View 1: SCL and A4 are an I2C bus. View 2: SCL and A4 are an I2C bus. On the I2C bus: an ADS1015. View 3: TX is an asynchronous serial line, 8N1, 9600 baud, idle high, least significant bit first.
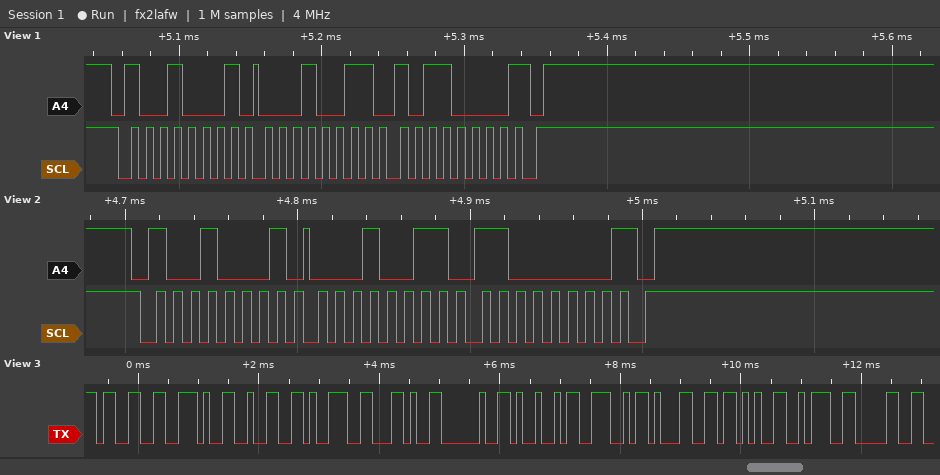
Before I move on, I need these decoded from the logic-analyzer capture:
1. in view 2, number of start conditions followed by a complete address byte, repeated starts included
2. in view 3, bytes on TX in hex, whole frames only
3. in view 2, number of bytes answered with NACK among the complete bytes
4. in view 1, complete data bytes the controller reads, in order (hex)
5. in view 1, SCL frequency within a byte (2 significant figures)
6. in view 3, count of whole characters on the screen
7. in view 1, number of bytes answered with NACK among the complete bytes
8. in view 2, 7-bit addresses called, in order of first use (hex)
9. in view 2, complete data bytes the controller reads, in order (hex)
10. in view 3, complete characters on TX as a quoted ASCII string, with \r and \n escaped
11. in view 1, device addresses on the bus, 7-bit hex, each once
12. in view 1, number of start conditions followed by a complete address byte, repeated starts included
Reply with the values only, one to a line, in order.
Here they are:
1
0x33 0x2E 0x32 0x39 0x2C 0x20 0x49 0x4E 0x31 0x2B 0x3A 0x30
1
13 B0
100 kHz
12
1
0x48
13 C0
"3.29, IN1+:0"
0x48
1
